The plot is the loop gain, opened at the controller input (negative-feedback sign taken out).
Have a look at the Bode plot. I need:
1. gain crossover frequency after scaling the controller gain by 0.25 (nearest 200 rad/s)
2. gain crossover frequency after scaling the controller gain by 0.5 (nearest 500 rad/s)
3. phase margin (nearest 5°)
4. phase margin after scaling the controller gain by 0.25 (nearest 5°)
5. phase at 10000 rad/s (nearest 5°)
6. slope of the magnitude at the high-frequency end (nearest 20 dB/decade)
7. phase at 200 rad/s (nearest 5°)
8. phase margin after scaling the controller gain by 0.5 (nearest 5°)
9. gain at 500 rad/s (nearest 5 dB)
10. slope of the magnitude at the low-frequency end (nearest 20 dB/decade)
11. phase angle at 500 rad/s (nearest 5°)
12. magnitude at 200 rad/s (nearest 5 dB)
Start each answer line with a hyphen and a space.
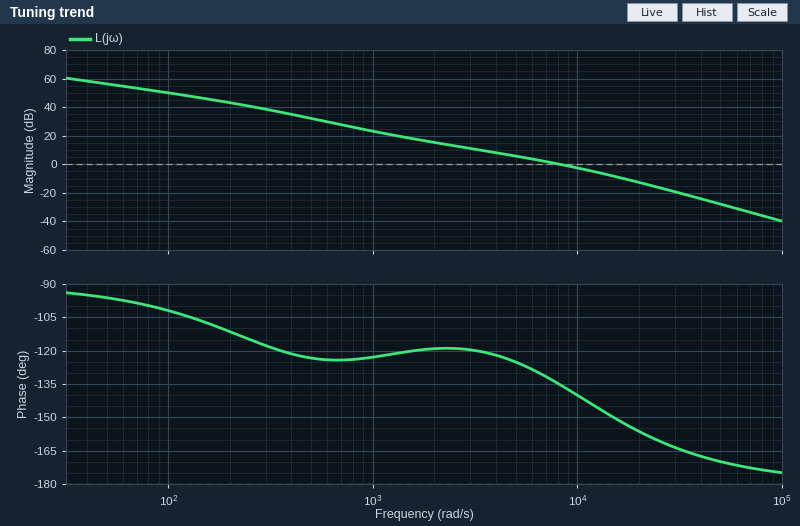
- 2800 rad/s
- 5000 rad/s
- 45°
- 60°
- -140°
- -40 dB/decade
- -110°
- 55°
- 30 dB
- -20 dB/decade
- -125°
- 45 dB
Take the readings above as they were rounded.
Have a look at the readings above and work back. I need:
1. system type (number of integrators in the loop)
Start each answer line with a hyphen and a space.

- 1
